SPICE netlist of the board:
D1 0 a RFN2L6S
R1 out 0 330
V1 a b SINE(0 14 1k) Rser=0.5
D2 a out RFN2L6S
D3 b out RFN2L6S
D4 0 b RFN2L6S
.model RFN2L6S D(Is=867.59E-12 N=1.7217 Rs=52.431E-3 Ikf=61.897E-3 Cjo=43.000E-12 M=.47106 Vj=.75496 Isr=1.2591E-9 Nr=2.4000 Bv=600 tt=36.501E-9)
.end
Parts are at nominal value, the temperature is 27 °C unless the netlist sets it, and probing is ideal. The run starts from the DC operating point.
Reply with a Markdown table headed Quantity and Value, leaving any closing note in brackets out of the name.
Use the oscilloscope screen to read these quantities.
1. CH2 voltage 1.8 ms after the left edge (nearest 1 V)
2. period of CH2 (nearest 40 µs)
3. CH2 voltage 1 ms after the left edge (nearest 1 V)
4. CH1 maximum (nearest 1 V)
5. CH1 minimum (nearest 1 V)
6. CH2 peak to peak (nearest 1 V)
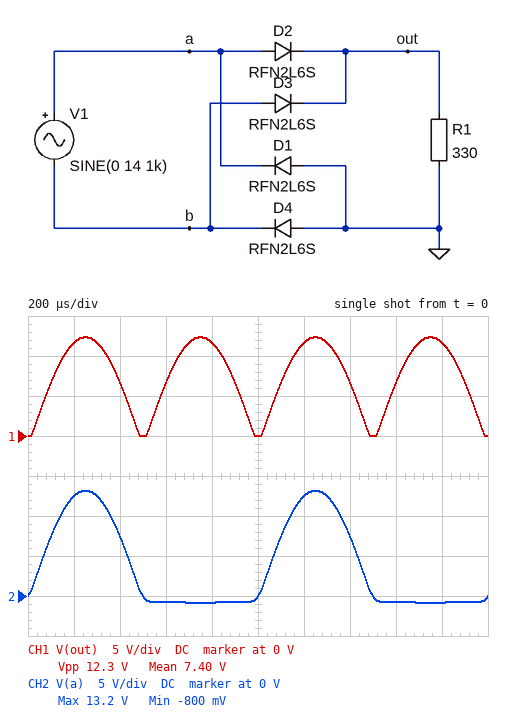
| Quantity | Value |
|---|---|
| CH2 voltage 1.8 ms after the left edge | -1 V |
| period of CH2 | 1.00 ms |
| CH2 voltage 1 ms after the left edge | 0 V |
| CH1 maximum | 12 V |
| CH1 minimum | 0 V |
| CH2 peak to peak | 14 V |
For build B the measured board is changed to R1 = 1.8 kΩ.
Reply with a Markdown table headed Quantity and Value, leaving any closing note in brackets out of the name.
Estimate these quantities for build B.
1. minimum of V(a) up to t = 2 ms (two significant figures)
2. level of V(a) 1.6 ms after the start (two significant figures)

| Quantity | Value |
|---|---|
| minimum of V(a) up to t = 2 ms | -720 mV |
| level of V(a) 1.6 ms after the start | -690 mV |
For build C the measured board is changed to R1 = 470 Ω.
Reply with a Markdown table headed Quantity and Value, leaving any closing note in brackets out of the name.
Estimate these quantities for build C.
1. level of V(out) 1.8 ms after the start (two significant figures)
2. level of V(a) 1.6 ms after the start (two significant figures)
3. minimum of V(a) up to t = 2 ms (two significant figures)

| Quantity | Value |
|---|---|
| level of V(out) 1.8 ms after the start | 12 V |
| level of V(a) 1.6 ms after the start | -760 mV |
| minimum of V(a) up to t = 2 ms | -800 mV |
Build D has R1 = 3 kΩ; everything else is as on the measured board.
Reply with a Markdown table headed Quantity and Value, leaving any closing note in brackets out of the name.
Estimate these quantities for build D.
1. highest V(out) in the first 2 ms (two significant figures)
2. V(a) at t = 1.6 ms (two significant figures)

| Quantity | Value |
|---|---|
| highest V(out) in the first 2 ms | 13 V |
| V(a) at t = 1.6 ms | -670 mV |
